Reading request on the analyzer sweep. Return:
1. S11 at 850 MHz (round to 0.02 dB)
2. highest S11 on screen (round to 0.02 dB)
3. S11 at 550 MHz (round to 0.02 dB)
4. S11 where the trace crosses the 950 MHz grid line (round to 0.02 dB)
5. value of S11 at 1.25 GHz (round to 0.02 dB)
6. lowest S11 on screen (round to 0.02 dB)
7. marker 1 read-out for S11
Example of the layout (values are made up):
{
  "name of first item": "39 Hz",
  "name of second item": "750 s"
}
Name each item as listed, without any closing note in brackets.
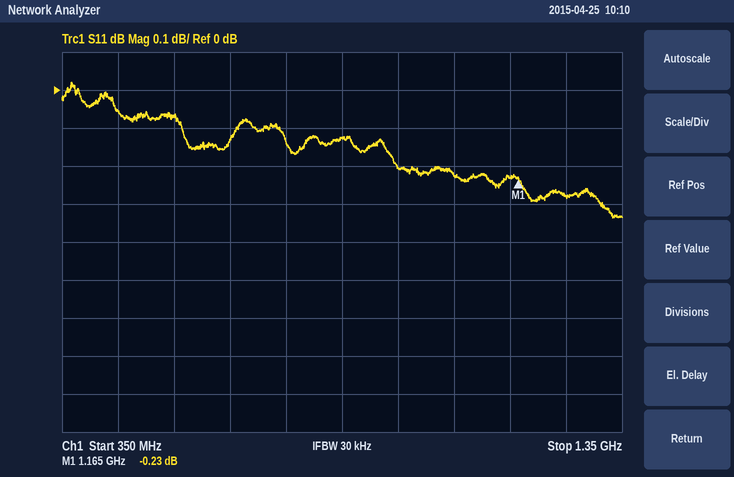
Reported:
{
  "S11 at 850 MHz": "-0.12 dB",
  "highest S11 on screen": "0.02 dB",
  "S11 at 550 MHz": "-0.06 dB",
  "S11 where the trace crosses the 950 MHz grid line": "-0.20 dB",
  "value of S11 at 1.25 GHz": "-0.28 dB",
  "lowest S11 on screen": "-0.34 dB",
  "marker 1 read-out for S11": "-0.23 dB"
}
